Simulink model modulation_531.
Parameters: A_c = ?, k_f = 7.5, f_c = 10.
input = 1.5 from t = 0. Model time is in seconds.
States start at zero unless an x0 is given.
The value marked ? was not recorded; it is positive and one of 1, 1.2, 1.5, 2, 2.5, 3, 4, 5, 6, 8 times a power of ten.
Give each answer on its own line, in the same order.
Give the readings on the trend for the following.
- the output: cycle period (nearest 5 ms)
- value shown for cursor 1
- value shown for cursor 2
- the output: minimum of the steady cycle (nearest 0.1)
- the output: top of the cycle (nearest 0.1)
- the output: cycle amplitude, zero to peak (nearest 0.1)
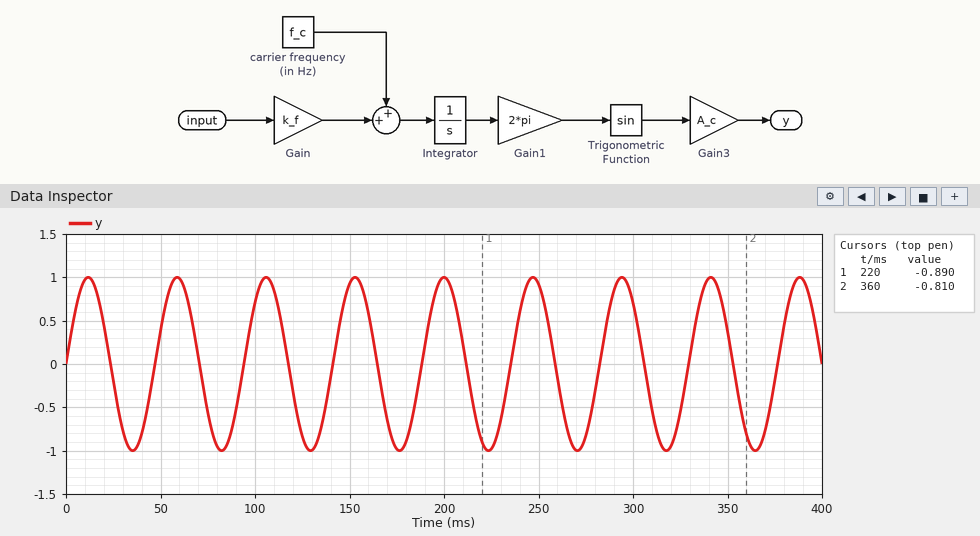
45 ms
-0.890
-0.810
-1.0
1.0
1.0
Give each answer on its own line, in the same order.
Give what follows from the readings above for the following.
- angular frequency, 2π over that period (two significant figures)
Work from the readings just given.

0.14 rad/ms
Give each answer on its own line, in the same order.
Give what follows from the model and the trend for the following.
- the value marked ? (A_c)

1
